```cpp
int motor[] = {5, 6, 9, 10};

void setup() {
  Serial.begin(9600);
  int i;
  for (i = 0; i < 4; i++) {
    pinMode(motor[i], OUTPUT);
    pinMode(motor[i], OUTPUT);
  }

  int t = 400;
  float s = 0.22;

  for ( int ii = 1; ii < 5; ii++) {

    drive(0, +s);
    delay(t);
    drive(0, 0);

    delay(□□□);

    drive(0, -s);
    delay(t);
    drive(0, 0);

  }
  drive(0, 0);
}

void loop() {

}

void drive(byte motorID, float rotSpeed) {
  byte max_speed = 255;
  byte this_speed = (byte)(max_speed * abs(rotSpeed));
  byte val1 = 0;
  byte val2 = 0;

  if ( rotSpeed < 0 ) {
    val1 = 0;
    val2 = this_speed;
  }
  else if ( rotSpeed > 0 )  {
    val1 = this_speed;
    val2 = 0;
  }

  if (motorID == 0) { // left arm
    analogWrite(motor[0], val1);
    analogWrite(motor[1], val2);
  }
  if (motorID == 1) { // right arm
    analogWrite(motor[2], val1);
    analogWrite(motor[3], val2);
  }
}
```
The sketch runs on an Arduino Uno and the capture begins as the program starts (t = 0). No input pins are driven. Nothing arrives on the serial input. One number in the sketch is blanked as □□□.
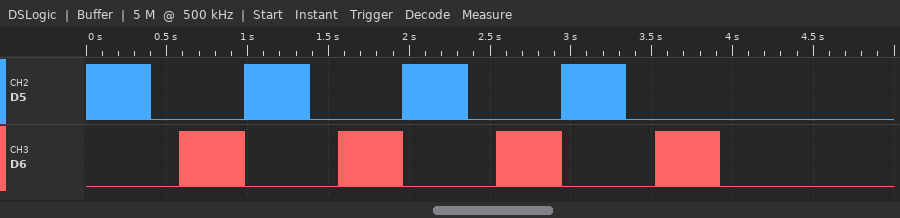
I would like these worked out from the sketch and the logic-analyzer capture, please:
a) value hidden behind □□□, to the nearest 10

180
